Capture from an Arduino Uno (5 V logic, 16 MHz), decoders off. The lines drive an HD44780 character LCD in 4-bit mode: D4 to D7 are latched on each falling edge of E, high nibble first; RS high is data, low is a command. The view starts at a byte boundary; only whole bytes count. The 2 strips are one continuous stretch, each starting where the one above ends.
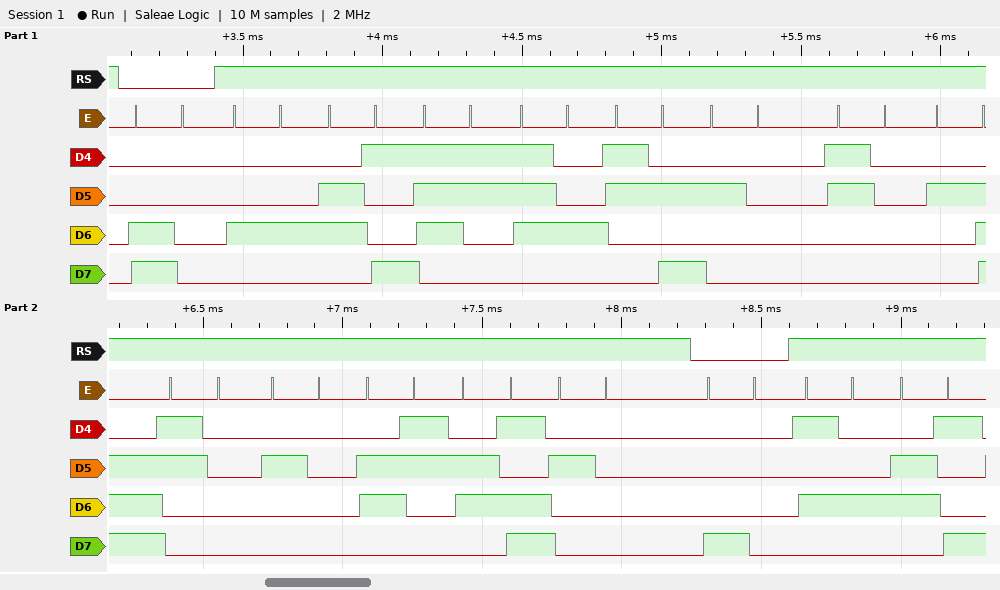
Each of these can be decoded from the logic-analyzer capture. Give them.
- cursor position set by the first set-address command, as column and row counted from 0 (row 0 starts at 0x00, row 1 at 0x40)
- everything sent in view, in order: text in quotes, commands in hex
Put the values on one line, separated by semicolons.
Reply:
column 0, row 1; 0xC0 "Dist: 0.0 cm " 0x80 "Ti"
